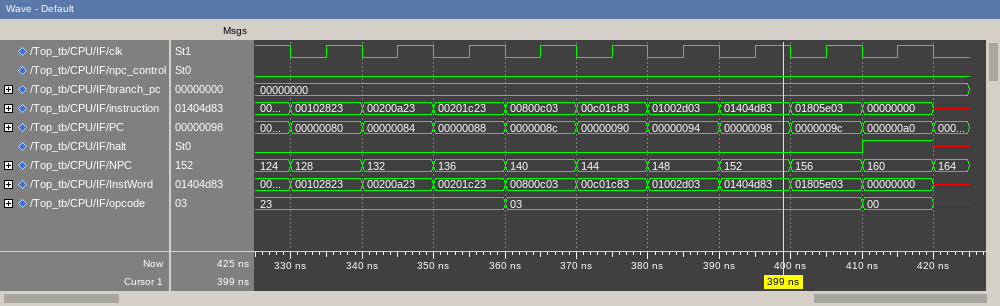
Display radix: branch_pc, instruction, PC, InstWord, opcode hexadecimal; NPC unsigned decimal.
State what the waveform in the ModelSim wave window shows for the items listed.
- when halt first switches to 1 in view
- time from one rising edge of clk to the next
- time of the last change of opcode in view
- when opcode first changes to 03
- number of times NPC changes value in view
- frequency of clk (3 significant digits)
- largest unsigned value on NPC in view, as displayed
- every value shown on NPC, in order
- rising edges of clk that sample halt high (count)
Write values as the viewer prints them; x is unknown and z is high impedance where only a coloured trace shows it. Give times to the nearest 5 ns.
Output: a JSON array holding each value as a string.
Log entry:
["410 ns", "10 ns", "420 ns", "360 ns", "10", "100 MHz", "164", "124, 128, 132, 136, 140, 144, 148, 152, 156, 160, 164", "1"]
